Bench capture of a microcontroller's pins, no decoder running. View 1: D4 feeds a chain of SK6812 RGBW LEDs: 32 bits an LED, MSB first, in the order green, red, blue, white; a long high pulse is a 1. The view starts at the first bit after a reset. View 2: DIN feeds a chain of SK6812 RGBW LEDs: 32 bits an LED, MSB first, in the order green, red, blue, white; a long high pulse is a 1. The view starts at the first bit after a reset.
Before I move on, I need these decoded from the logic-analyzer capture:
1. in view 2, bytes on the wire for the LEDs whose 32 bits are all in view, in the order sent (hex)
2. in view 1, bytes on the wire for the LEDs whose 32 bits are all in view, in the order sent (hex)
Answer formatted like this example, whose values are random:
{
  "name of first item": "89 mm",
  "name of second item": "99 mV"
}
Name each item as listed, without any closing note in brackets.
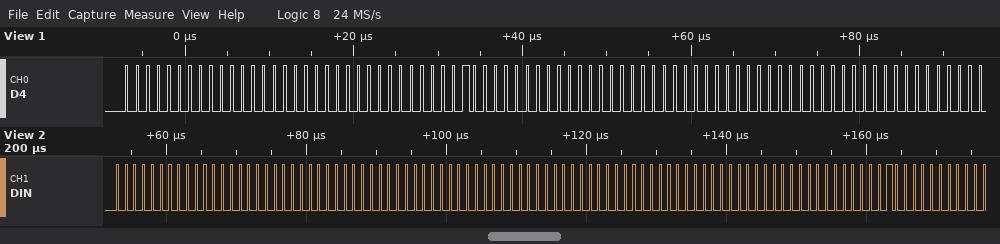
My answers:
{
  "in view 2, bytes on the wire for the LEDs whose 32 bits are all in view, in the order sent": "00 00 00 00 00 00 00 00 00 00 00 80",
  "in view 1, bytes on the wire for the LEDs whose 32 bits are all in view, in the order sent": "00 00 00 00 80 00 00 00"
}
